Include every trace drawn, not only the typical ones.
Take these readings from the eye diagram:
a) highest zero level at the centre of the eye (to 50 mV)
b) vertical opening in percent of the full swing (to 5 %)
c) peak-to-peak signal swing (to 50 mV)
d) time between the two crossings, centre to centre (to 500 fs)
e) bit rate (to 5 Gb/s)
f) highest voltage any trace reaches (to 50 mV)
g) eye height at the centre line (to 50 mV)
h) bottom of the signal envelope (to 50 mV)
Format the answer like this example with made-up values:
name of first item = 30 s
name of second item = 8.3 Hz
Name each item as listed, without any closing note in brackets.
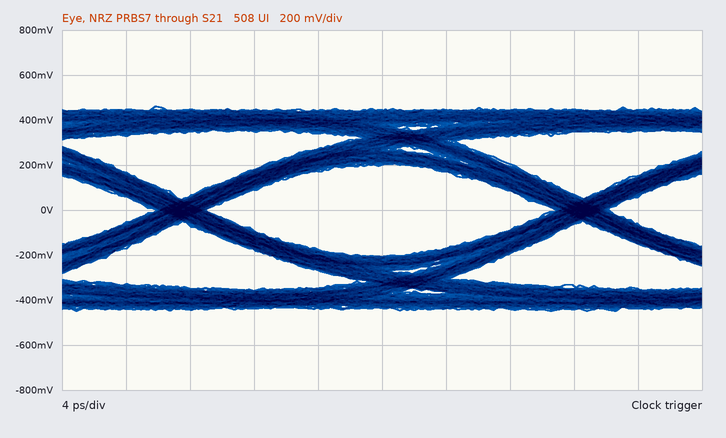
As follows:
highest zero level at the centre of the eye = -200 mV
vertical opening in percent of the full swing = 45 %
peak-to-peak signal swing = 900 mV
time between the two crossings, centre to centre = 25.0 ps
bit rate = 40 Gb/s
highest voltage any trace reaches = 450 mV
eye height at the centre line = 400 mV
bottom of the signal envelope = -450 mV
